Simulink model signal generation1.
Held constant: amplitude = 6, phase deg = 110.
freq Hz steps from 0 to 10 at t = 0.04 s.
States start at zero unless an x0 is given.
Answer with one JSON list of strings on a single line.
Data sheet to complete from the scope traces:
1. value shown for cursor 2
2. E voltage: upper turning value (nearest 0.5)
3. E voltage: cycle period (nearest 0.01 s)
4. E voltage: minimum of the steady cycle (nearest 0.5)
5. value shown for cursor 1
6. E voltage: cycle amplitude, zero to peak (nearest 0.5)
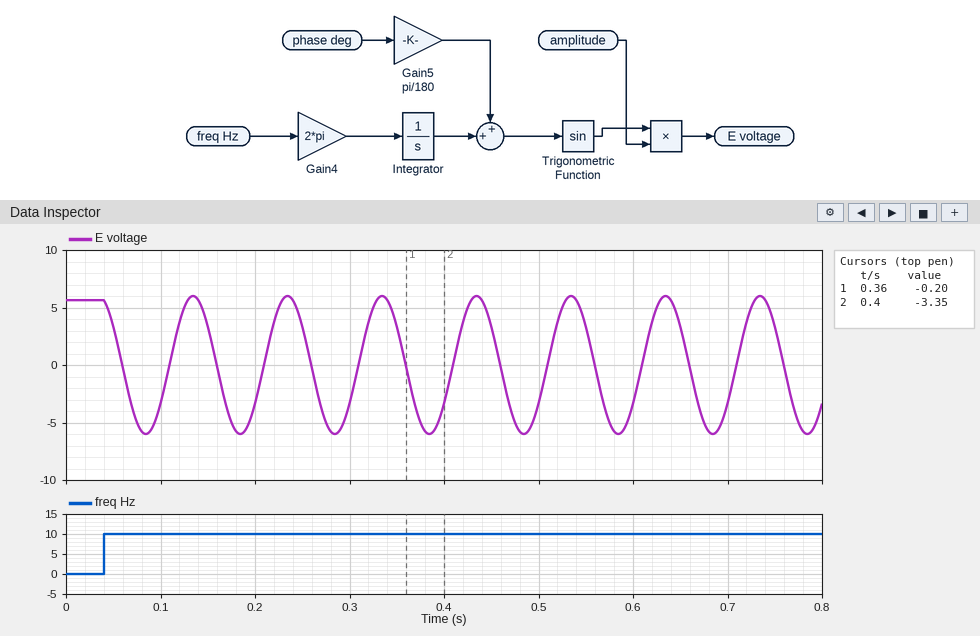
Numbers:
["-3.35", "6.0", "0.10 s", "-6.0", "-0.20", "6.0"]
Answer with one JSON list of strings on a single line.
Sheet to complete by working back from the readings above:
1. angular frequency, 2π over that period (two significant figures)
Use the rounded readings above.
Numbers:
["63 rad/s"]
